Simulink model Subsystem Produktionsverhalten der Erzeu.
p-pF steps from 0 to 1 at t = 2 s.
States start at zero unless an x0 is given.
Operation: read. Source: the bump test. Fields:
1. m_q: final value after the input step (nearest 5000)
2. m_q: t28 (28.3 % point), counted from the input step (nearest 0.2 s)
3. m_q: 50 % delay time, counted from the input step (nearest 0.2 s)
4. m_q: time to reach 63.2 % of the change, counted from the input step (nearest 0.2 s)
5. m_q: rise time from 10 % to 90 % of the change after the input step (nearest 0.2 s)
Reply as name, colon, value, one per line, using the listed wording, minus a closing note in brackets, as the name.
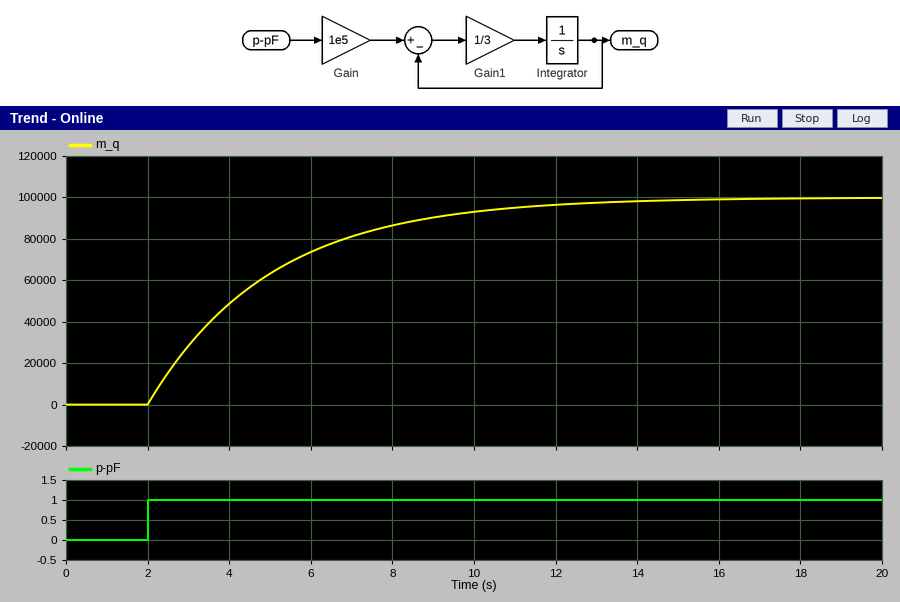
m_q: final value after the input step: 100000
m_q: t28 (28.3 % point), counted from the input step: 1.0 s
m_q: 50 % delay time, counted from the input step: 2.0 s
m_q: time to reach 63.2 % of the change, counted from the input step: 3.0 s
m_q: rise time from 10 % to 90 % of the change after the input step: 6.6 s
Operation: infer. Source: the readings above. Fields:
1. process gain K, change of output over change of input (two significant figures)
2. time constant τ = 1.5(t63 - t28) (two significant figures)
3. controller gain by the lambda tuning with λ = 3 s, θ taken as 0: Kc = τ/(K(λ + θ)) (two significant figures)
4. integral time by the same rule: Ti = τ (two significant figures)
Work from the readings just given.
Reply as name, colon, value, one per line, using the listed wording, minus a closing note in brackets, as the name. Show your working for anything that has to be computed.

process gain K, change of output over change of input: (100000 - 0) / 1 = 100000
time constant τ = 1.5(t63 - t28): 1.5 × (3 - 1) = 3.0 s
controller gain by the lambda tuning with λ = 3 s, θ taken as 0: Kc = τ/(K(λ + θ)): 3 / (100000 × (3 + 0)) = 0.000010
integral time by the same rule: Ti = τ: 3.0 s
